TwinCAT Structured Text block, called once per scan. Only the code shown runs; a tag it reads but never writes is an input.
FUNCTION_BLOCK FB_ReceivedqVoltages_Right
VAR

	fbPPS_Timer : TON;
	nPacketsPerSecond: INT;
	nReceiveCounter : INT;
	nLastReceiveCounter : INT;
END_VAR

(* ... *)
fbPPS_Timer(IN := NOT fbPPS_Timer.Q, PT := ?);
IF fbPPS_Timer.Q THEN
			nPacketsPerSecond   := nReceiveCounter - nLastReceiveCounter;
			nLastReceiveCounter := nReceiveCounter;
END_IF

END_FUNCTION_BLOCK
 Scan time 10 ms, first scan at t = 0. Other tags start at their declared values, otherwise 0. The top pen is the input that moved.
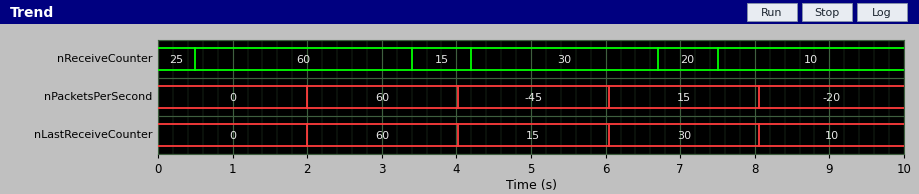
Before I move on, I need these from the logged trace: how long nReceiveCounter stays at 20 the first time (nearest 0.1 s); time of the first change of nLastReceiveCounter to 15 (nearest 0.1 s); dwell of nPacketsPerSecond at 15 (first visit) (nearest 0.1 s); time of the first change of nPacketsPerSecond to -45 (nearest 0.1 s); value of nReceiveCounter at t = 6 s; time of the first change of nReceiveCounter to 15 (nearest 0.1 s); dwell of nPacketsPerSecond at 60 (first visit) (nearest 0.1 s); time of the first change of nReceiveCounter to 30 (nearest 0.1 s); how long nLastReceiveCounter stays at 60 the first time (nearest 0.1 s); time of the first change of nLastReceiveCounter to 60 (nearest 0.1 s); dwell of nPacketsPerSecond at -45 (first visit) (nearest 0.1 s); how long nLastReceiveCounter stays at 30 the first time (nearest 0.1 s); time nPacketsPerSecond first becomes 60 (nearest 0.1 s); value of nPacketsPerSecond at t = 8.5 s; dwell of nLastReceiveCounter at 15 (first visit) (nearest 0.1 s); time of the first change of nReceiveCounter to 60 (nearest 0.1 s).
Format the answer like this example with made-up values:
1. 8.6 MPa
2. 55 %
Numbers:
1. 0.8 s
2. 4.0 s
3. 2.0 s
4. 4.0 s
5. 30
6. 3.4 s
7. 2.0 s
8. 4.2 s
9. 2.0 s
10. 2.0 s
11. 2.0 s
12. 2.0 s
13. 2.0 s
14. -20
15. 2.0 s
16. 0.5 s
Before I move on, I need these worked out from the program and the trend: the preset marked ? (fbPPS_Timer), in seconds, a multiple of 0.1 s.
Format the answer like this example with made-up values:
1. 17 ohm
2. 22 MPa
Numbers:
1. 2.0 s
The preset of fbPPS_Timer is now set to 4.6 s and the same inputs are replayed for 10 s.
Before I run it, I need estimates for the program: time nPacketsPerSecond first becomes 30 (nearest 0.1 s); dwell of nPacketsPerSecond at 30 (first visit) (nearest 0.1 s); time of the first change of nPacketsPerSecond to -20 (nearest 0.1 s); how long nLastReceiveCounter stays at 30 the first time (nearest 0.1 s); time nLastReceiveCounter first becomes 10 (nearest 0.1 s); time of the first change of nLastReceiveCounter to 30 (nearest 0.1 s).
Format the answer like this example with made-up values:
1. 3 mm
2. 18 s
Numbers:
1. 4.6 s
2. 4.6 s
3. 9.2 s
4. 4.6 s
5. 9.2 s
6. 4.6 s
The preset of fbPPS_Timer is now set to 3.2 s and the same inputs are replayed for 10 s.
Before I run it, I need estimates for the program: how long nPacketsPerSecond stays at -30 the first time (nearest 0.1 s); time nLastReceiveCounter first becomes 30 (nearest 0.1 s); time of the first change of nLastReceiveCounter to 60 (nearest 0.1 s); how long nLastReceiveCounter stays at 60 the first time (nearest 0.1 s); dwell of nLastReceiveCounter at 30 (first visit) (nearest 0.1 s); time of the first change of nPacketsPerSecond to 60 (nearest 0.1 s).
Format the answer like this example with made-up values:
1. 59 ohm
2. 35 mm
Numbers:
1. 3.2 s
2. 6.4 s
3. 3.2 s
4. 3.2 s
5. 3.2 s
6. 3.2 s
